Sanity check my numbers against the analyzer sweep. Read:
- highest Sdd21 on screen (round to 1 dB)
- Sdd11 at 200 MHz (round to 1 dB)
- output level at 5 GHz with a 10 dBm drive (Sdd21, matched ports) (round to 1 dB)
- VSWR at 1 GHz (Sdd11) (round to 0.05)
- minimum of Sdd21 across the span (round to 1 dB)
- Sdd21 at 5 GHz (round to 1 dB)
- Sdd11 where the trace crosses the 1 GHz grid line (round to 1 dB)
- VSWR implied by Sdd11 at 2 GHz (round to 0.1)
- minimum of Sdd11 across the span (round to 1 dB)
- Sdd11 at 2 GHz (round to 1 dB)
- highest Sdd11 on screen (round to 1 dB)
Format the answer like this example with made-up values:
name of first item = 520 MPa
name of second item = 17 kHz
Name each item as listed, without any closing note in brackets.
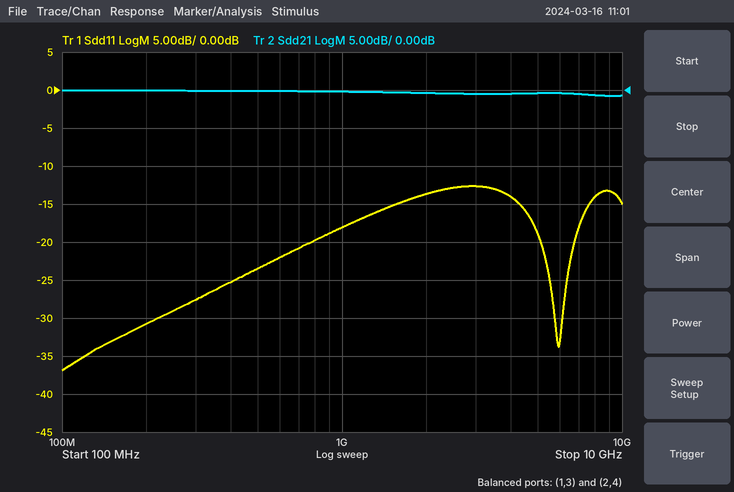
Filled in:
highest Sdd21 on screen = 0 dB
Sdd11 at 200 MHz = -31 dB
output level at 5 GHz with a 10 dBm drive (Sdd21, matched ports) = 10 dBm
VSWR at 1 GHz (Sdd11) = 1.30
minimum of Sdd21 across the span = -1 dB
Sdd21 at 5 GHz = 0 dB
Sdd11 where the trace crosses the 1 GHz grid line = -18 dB
VSWR implied by Sdd11 at 2 GHz = 1.5
minimum of Sdd11 across the span = -37 dB
Sdd11 at 2 GHz = -14 dB
highest Sdd11 on screen = -13 dB
